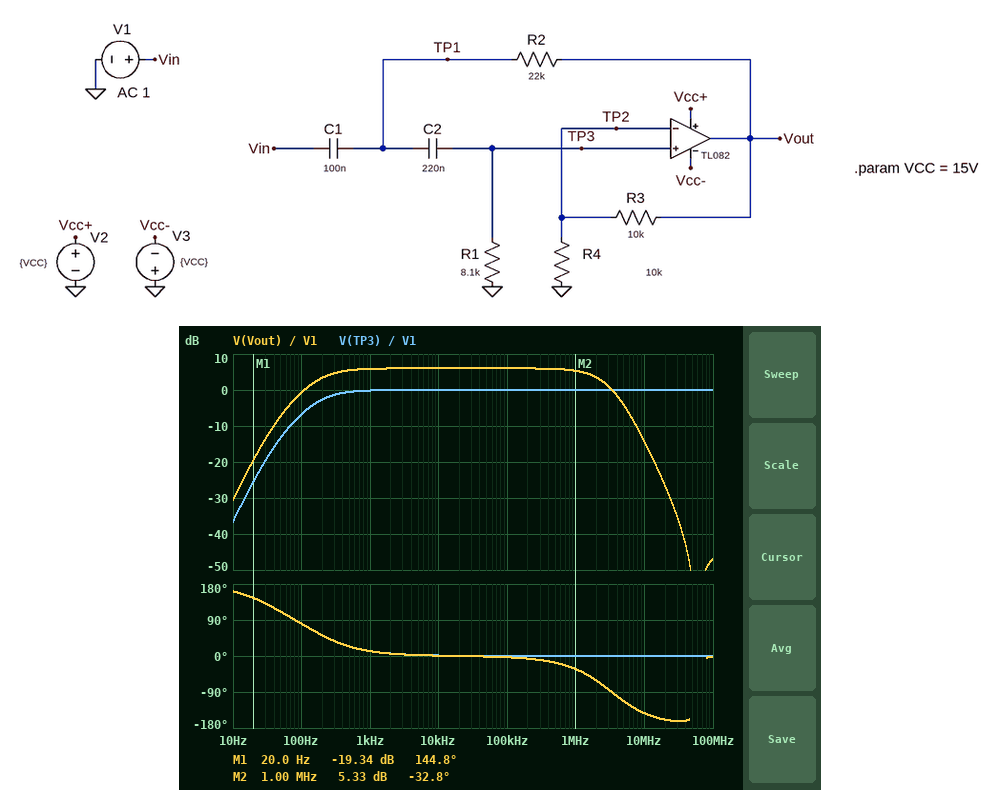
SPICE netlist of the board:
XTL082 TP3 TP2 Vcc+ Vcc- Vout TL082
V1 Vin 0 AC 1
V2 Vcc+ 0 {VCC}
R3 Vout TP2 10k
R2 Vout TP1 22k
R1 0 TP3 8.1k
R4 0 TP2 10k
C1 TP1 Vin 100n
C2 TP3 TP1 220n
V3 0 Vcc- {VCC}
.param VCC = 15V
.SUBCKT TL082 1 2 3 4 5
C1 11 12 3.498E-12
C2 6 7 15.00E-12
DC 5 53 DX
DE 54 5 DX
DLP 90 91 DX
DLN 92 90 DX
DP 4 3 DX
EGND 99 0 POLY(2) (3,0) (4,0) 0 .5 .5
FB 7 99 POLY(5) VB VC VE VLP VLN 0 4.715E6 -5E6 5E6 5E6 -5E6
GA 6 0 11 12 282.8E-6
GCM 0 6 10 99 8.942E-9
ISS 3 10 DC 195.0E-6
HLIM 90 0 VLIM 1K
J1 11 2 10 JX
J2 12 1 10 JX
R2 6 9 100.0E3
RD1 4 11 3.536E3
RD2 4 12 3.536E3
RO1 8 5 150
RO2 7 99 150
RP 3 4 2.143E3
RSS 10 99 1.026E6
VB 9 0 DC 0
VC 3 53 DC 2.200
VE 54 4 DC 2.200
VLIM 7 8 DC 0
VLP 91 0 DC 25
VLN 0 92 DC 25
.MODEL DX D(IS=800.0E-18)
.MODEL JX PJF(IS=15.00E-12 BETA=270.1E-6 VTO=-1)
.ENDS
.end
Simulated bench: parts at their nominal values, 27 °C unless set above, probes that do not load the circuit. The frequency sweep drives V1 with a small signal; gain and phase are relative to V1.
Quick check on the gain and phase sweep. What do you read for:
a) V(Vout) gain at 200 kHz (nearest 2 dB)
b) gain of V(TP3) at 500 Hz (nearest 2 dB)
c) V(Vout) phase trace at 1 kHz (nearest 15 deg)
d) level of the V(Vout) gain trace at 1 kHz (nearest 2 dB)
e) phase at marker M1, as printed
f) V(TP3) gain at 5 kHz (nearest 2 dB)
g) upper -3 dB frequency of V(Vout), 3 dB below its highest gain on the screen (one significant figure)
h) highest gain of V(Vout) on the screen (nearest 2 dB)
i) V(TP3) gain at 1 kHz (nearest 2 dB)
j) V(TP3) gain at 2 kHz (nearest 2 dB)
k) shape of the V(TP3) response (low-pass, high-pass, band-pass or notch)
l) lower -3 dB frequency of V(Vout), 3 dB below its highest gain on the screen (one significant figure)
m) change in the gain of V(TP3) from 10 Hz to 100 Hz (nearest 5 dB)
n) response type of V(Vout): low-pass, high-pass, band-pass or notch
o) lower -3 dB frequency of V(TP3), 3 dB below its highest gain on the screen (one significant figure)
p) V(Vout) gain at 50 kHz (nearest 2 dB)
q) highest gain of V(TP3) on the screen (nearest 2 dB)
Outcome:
6 dB
0 dB
15 deg
6 dB
144.8 deg
0 dB
2 MHz
6 dB
0 dB
0 dB
high-pass
200 Hz
30 dB
band-pass
200 Hz
6 dB
0 dB
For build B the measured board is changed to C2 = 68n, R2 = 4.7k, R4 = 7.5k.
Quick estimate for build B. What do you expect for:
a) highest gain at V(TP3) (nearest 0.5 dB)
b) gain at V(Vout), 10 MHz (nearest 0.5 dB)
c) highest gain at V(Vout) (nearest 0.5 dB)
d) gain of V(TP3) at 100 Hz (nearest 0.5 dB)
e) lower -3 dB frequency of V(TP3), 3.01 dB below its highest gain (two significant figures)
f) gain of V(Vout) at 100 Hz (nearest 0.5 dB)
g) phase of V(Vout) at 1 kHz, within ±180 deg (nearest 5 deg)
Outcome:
19.5 dB
-15.5 dB
26.5 dB
-19.0 dB
300 Hz
-11.5 dB
0 deg
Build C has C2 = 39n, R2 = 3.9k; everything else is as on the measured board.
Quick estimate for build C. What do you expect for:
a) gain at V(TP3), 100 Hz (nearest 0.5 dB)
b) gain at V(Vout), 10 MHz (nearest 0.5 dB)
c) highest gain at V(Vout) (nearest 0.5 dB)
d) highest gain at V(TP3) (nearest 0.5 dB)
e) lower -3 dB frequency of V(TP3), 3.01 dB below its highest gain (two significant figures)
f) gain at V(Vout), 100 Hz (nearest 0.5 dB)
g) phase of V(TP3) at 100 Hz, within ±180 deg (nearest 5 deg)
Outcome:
-26.0 dB
-16.0 dB
10.5 dB
4.5 dB
380 Hz
-20.0 dB
170 deg
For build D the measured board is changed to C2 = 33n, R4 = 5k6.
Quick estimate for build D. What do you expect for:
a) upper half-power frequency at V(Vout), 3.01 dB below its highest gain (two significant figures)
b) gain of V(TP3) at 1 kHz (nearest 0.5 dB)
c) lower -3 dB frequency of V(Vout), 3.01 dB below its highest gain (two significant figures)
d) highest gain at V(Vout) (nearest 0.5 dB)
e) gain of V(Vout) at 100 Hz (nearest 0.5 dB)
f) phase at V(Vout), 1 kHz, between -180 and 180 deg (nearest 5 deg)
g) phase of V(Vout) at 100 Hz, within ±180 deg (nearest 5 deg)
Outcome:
1.5 MHz
-1.5 dB
600 Hz
9.0 dB
-8.5 dB
35 deg
115 deg
